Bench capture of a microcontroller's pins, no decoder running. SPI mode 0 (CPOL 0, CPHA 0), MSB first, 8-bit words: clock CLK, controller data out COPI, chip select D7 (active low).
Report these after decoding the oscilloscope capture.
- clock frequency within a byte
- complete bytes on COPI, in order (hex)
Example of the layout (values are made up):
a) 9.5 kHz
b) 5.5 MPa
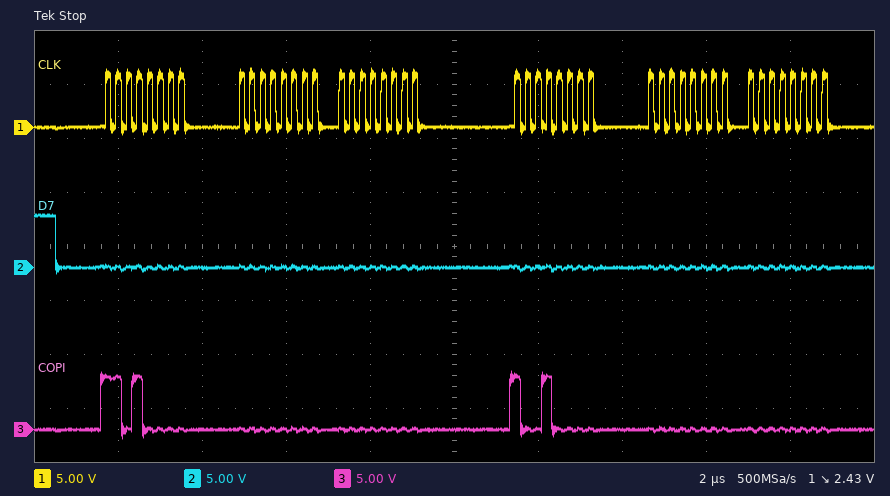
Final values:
a) 4 MHz
b) 0xD0 0x00 0x00 0x90 0x00 0x00
